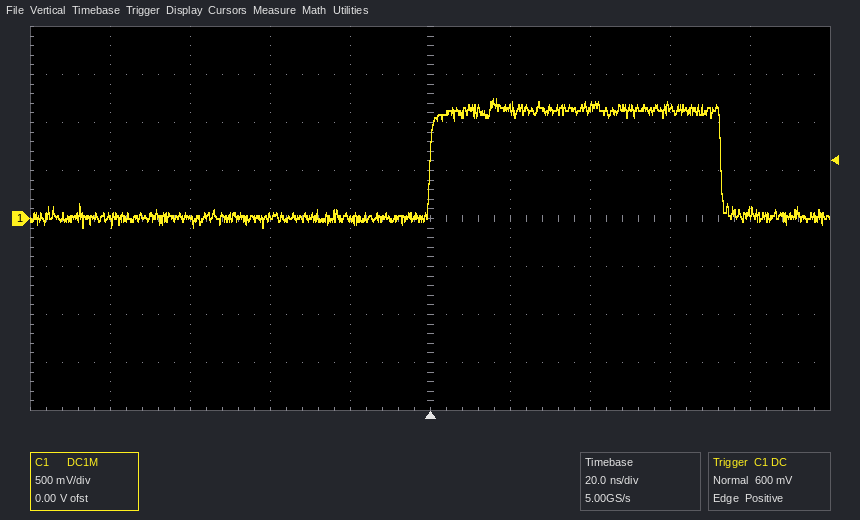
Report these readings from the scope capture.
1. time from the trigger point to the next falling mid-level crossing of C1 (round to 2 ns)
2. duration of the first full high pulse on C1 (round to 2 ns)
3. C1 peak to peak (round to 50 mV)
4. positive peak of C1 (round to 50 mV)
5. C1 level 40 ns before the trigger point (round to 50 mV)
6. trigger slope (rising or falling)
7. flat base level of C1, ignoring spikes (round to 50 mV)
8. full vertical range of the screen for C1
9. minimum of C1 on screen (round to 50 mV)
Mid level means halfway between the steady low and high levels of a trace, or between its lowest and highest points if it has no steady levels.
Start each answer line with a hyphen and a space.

- 72 ns
- 72 ns
- 1.35 V
- 1.25 V
- 0 mV
- rising
- 0 mV
- 4 V
- -100 mV
